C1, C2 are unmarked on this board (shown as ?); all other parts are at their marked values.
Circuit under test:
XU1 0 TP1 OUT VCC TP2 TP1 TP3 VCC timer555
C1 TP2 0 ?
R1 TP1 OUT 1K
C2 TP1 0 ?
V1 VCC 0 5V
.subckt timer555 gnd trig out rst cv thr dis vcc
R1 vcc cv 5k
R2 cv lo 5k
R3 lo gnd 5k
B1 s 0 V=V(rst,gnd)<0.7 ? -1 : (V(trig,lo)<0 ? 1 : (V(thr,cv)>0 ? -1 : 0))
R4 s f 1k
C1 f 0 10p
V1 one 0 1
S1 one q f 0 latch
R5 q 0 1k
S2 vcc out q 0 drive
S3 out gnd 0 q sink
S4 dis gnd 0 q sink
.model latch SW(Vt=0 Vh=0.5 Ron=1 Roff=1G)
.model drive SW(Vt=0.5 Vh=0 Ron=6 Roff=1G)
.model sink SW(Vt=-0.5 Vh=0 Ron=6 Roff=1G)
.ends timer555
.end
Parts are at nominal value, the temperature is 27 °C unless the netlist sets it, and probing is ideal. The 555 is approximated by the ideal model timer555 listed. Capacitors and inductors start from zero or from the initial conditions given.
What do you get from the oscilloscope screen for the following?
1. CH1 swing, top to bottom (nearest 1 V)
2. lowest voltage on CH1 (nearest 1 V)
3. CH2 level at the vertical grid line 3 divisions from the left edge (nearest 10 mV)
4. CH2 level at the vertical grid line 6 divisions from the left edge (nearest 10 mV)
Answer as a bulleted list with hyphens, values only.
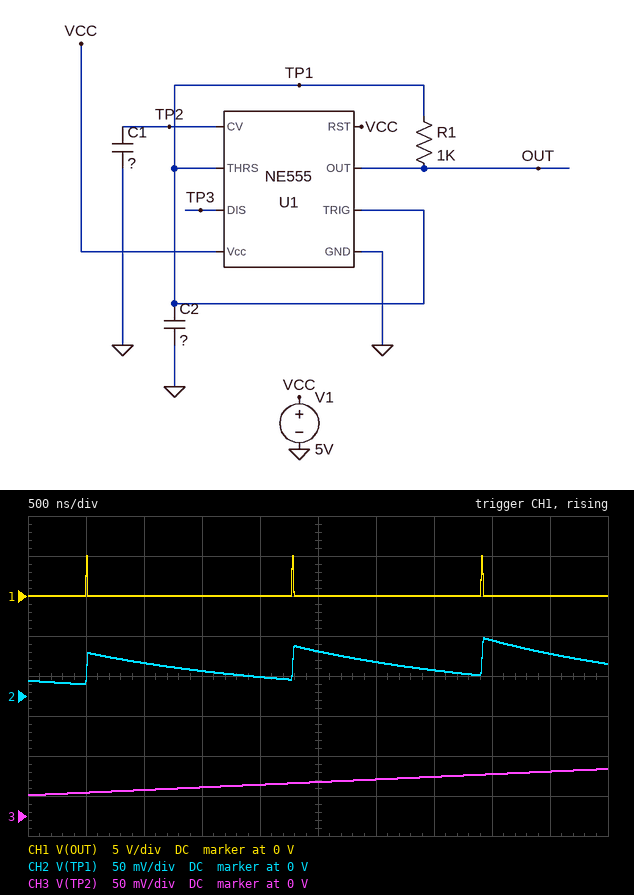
- 5 V
- 0 V
- 30 mV
- 40 mV
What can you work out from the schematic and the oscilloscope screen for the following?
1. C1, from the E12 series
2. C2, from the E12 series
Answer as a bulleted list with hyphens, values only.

- 150 nF
- 1.8 nF
